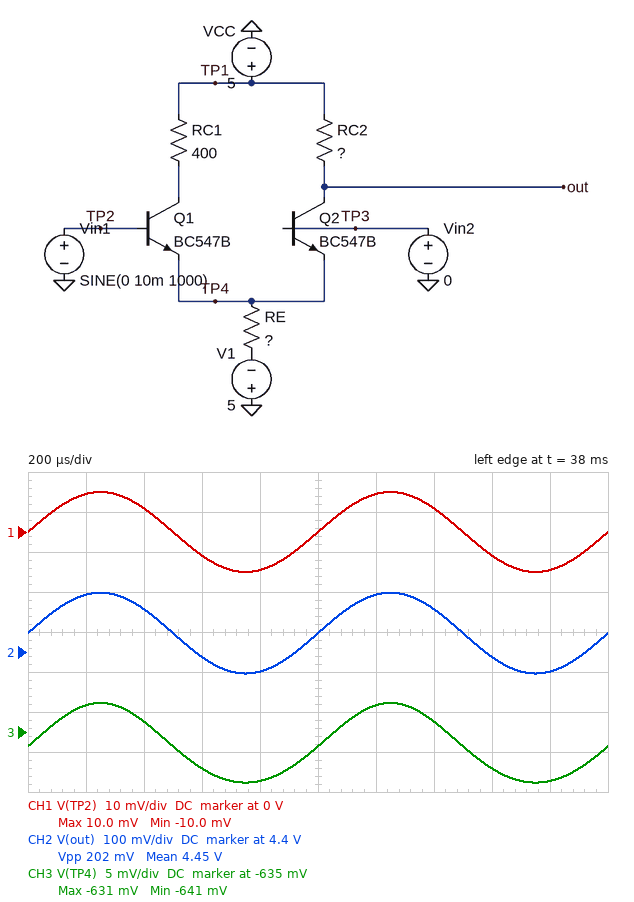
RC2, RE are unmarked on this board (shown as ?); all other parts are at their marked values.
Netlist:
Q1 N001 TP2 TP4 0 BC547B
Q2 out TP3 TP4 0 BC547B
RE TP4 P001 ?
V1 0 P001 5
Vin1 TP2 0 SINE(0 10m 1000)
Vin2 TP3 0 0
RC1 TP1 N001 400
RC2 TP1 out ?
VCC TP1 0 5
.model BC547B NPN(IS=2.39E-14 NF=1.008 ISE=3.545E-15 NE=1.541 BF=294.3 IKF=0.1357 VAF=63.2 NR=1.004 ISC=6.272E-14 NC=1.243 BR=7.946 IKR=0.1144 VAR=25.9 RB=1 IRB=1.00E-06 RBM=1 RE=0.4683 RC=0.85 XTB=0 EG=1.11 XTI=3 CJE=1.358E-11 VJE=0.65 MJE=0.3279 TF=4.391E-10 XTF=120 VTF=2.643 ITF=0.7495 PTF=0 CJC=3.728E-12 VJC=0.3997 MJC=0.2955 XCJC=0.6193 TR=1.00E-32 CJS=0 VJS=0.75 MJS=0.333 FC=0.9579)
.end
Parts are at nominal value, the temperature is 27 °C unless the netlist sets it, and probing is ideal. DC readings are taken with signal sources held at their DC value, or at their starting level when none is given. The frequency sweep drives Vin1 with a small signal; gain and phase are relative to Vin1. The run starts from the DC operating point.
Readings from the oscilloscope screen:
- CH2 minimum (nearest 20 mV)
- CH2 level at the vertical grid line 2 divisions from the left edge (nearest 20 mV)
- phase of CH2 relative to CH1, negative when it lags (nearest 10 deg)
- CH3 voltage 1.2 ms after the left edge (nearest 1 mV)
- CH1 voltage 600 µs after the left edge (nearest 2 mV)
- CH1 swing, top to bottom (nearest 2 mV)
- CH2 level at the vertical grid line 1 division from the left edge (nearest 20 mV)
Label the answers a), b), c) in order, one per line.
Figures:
a) 4.34 V
b) 4.50 V
c) 0 deg
d) -632 mV
e) -6 mV
f) 20 mV
g) 4.54 V
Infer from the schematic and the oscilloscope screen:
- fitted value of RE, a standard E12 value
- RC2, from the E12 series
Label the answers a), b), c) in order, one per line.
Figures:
a) 2.2 kΩ
b) 560 Ω
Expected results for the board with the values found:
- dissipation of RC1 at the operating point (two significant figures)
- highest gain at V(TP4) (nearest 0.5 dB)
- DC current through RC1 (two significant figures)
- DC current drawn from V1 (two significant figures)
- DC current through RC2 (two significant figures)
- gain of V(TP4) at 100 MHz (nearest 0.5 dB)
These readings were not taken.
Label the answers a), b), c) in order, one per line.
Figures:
a) 390 µW
b) -6.0 dB
c) 990 µA
d) 2.0 mA
e) 990 µA
f) -6.0 dB
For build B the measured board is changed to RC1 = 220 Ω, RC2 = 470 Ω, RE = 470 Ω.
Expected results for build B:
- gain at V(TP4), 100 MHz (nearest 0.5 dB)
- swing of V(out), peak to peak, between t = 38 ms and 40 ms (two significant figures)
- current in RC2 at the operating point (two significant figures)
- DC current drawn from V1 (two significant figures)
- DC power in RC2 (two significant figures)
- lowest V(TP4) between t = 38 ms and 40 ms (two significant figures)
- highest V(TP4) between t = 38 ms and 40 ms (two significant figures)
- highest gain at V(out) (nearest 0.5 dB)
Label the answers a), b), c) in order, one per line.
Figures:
a) -6.0 dB
b) 710 mV
c) 4.5 mA
d) 9.2 mA
e) 9.7 mW
f) -680 mV
g) -670 mV
h) 31.0 dB
